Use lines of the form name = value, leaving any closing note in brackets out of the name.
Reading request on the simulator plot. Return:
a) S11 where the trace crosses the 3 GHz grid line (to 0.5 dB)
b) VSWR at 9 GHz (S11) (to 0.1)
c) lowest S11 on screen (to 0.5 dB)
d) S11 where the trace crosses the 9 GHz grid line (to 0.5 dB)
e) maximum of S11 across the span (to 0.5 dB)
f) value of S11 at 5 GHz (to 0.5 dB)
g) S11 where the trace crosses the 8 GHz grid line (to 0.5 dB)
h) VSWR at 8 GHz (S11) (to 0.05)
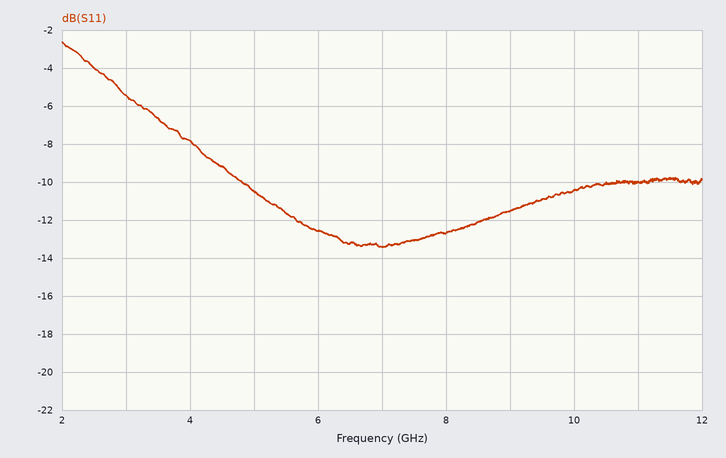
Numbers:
S11 where the trace crosses the 3 GHz grid line = -5.5 dB
VSWR at 9 GHz (S11) = 1.7
lowest S11 on screen = -13.5 dB
S11 where the trace crosses the 9 GHz grid line = -11.5 dB
maximum of S11 across the span = -2.5 dB
value of S11 at 5 GHz = -10.5 dB
S11 where the trace crosses the 8 GHz grid line = -12.5 dB
VSWR at 8 GHz (S11) = 1.60
